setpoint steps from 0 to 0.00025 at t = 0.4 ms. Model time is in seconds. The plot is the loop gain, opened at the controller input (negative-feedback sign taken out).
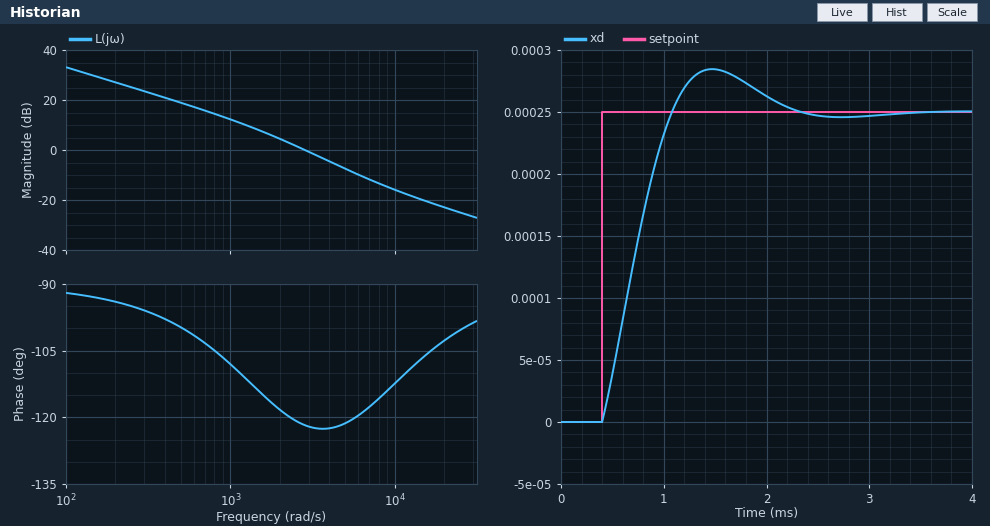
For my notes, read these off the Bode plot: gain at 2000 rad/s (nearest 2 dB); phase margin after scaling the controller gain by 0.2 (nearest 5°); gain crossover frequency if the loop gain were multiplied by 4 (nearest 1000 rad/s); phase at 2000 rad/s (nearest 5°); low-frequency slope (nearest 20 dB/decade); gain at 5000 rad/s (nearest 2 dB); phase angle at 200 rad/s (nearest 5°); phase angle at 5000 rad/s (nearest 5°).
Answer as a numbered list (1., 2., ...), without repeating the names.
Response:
1. 4 dB
2. 75°
3. 7000 rad/s
4. -120°
5. -20 dB/decade
6. -8 dB
7. -95°
8. -120°
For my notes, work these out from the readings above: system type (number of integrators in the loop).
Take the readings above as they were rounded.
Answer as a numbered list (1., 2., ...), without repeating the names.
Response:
1. 1
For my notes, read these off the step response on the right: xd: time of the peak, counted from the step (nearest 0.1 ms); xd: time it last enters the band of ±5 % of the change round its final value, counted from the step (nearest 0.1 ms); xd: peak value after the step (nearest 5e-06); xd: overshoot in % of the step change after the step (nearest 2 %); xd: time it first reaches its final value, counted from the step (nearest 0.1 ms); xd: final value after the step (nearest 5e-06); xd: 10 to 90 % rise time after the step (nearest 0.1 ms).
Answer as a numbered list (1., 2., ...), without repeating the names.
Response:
1. 1.1 ms
2. 1.6 ms
3. 0.000285
4. 14 %
5. 0.7 ms
6. 0.000250
7. 0.5 ms
